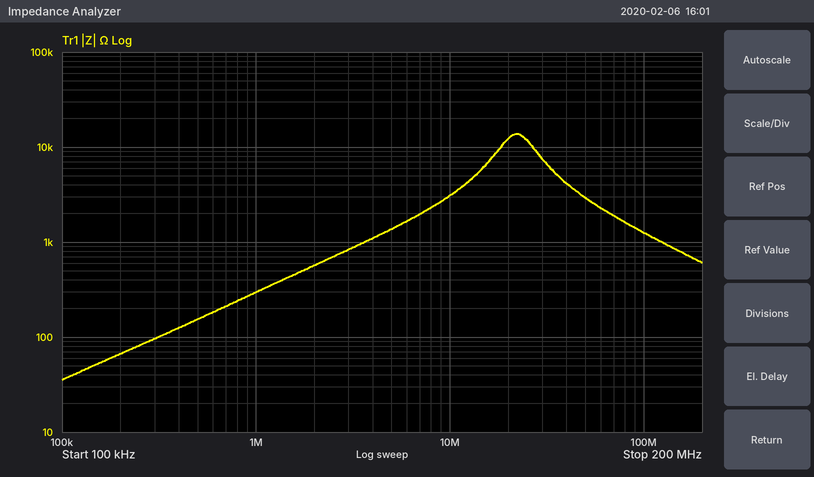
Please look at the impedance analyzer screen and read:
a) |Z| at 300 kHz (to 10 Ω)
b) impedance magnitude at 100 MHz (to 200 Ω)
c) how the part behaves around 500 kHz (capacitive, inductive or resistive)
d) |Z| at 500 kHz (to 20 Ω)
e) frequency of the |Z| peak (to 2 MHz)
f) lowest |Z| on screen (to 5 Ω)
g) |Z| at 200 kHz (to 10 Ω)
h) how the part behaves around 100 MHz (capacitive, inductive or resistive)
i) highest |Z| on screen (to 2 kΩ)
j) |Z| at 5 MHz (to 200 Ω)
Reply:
100 Ω
1.2 kΩ
inductive
160 Ω
22 MHz
35 Ω
70 Ω
capacitive
14 kΩ
1.4 kΩ
